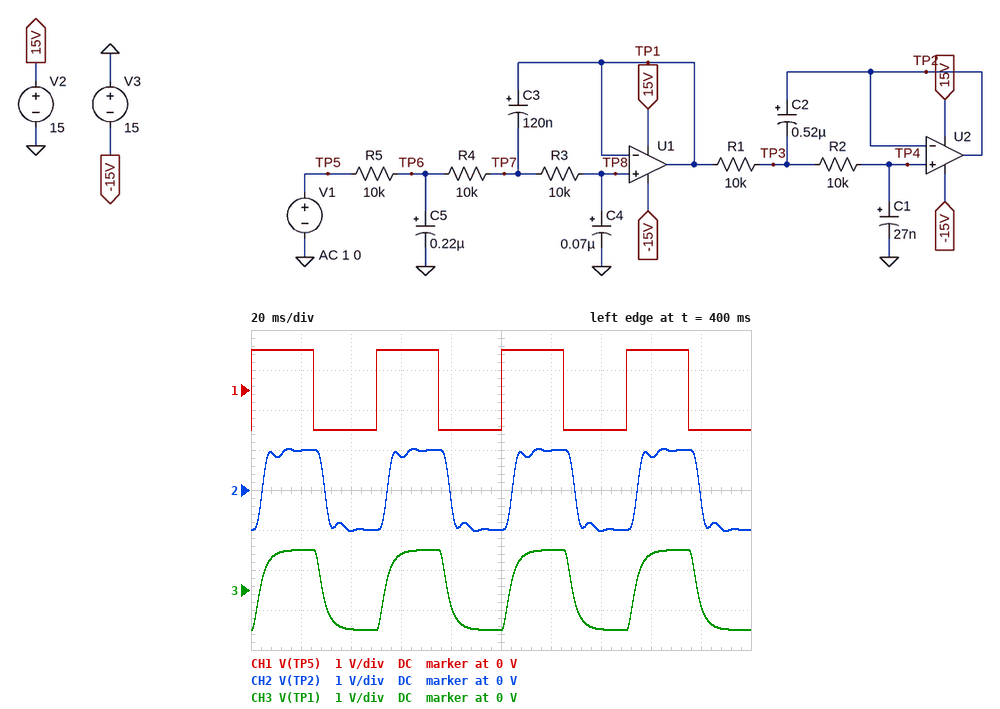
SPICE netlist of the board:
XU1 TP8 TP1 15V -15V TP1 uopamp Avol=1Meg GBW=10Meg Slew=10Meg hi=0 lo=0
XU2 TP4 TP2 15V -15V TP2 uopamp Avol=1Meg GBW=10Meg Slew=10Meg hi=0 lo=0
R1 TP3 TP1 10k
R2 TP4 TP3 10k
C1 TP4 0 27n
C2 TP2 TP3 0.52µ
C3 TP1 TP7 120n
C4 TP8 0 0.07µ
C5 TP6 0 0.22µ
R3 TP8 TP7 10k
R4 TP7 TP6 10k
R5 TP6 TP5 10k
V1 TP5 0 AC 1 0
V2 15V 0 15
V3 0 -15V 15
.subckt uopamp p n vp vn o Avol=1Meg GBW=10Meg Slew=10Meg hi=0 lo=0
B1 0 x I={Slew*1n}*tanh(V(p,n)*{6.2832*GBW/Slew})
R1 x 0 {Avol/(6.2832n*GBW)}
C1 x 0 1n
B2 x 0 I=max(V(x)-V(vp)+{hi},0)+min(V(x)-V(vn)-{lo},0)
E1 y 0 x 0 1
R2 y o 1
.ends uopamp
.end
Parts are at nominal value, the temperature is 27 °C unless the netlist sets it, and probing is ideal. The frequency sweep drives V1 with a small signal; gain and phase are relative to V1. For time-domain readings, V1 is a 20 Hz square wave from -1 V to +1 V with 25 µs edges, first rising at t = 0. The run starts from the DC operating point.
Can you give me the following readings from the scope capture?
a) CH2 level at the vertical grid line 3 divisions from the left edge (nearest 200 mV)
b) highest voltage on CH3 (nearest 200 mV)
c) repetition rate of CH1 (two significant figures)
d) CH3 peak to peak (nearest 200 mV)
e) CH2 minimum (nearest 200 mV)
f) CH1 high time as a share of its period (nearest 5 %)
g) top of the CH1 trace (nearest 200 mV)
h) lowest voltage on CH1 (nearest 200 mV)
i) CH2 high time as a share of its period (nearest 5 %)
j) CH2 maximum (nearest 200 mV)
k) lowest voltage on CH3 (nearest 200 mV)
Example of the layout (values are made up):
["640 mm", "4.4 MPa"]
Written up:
["800 mV", "1.0 V", "20 Hz", "2.0 V", "-1.0 V", "50 %", "1.0 V", "-1.0 V", "50 %", "1.0 V", "-1.0 V"]
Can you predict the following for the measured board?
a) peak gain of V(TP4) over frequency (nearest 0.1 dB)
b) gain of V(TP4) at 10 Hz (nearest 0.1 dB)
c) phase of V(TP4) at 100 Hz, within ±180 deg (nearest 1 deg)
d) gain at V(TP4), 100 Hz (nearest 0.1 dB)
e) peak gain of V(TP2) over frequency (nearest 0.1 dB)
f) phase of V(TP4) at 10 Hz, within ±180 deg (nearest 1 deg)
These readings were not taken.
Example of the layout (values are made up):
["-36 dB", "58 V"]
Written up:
["0 dB", "-0.1 dB", "-149 deg", "-2.6 dB", "0 dB", "-17 deg"]
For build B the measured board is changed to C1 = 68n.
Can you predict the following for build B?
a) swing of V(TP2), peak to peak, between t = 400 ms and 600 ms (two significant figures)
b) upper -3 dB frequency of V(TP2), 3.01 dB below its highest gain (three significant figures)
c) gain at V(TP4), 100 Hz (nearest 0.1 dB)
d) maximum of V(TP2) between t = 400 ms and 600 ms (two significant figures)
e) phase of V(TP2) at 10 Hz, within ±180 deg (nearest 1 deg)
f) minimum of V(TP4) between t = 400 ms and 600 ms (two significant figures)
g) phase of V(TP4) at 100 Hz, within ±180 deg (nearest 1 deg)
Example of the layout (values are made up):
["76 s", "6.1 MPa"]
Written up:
["2.3 V", "82.7 Hz", "-7.1 dB", "1.1 V", "-20 deg", "-1.1 V", "134 deg"]
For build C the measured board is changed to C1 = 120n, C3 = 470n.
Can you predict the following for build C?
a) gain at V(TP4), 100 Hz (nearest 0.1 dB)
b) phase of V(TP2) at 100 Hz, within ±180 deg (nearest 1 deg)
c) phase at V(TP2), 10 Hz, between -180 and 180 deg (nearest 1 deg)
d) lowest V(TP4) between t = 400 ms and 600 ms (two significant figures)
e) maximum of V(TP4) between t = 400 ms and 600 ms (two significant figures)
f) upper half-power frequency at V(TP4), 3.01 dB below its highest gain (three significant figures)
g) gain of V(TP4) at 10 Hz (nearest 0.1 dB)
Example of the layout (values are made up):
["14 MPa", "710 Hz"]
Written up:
["-15.9 dB", "64 deg", "-24 deg", "-1.4 V", "1.4 V", "62.3 Hz", "0.1 dB"]
